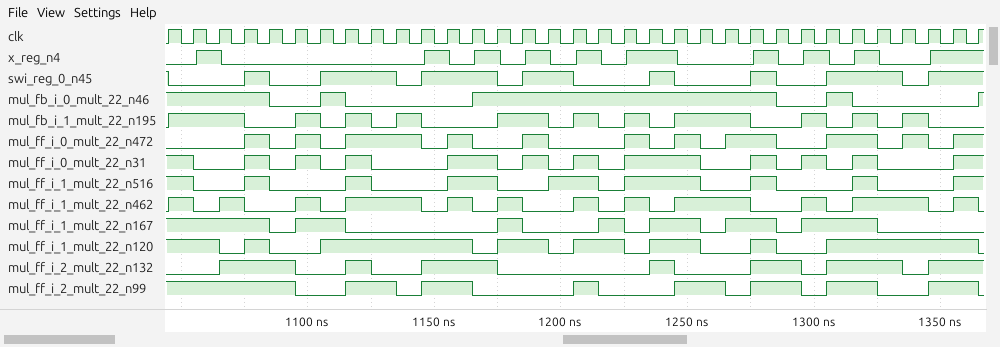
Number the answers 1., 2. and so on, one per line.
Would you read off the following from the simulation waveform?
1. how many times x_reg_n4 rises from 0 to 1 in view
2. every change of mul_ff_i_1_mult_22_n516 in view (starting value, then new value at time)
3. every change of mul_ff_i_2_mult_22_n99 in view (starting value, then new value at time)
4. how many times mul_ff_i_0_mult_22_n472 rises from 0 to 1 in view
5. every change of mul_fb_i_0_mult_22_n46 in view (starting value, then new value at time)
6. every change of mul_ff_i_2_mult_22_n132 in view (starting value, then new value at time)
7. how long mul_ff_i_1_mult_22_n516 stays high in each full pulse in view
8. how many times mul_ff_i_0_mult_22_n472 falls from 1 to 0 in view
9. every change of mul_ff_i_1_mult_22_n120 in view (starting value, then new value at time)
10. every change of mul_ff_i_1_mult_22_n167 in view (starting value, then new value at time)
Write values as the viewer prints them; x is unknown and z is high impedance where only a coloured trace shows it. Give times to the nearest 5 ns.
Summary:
1. 10
2. 1, 0 at 1055 ns, 1 at 1075 ns, 0 at 1085 ns, 1 at 1115 ns, 0 at 1125 ns, 1 at 1155 ns, 0 at 1175 ns, 1 at 1195 ns, 0 at 1215 ns, 1 at 1225 ns, 0 at 1255 ns, 1 at 1275 ns, 0 at 1285 ns, 1 at 1315 ns, 0 at 1325 ns, 1 at 1355 ns
3. 1, 0 at 1095 ns, 1 at 1115 ns, 0 at 1135 ns, 1 at 1145 ns, 0 at 1165 ns, 1 at 1205 ns, 0 at 1215 ns, 1 at 1245 ns, 0 at 1265 ns, 1 at 1275 ns, 0 at 1295 ns, 1 at 1305 ns, 0 at 1325 ns, 1 at 1345 ns, 0 at 1365 ns
4. 11
5. 1, 0 at 1085 ns, 1 at 1105 ns, 0 at 1115 ns, 1 at 1165 ns, 0 at 1285 ns, 1 at 1305 ns, 0 at 1315 ns, 1 at 1365 ns
6. 0, 1 at 1065 ns, 0 at 1095 ns, 1 at 1115 ns, 0 at 1125 ns, 1 at 1145 ns, 0 at 1175 ns, 1 at 1235 ns, 0 at 1245 ns, 1 at 1275 ns, 0 at 1295 ns, 1 at 1305 ns, 0 at 1335 ns, 1 at 1345 ns
7. 10 ns, 10 ns, 20 ns, 20 ns, 30 ns, 10 ns, 10 ns
8. 10
9. 1, 0 at 1065 ns, 1 at 1075 ns, 0 at 1085 ns, 1 at 1105 ns, 0 at 1165 ns, 1 at 1175 ns, 0 at 1195 ns, 1 at 1205 ns, 0 at 1225 ns, 1 at 1235 ns, 0 at 1255 ns, 1 at 1275 ns, 0 at 1285 ns, 1 at 1305 ns, 0 at 1365 ns
10. 1, 0 at 1085 ns, 1 at 1095 ns, 0 at 1115 ns, 1 at 1175 ns, 0 at 1185 ns, 1 at 1215 ns, 0 at 1225 ns, 1 at 1235 ns, 0 at 1255 ns, 1 at 1265 ns, 0 at 1285 ns, 1 at 1295 ns, 0 at 1325 ns
